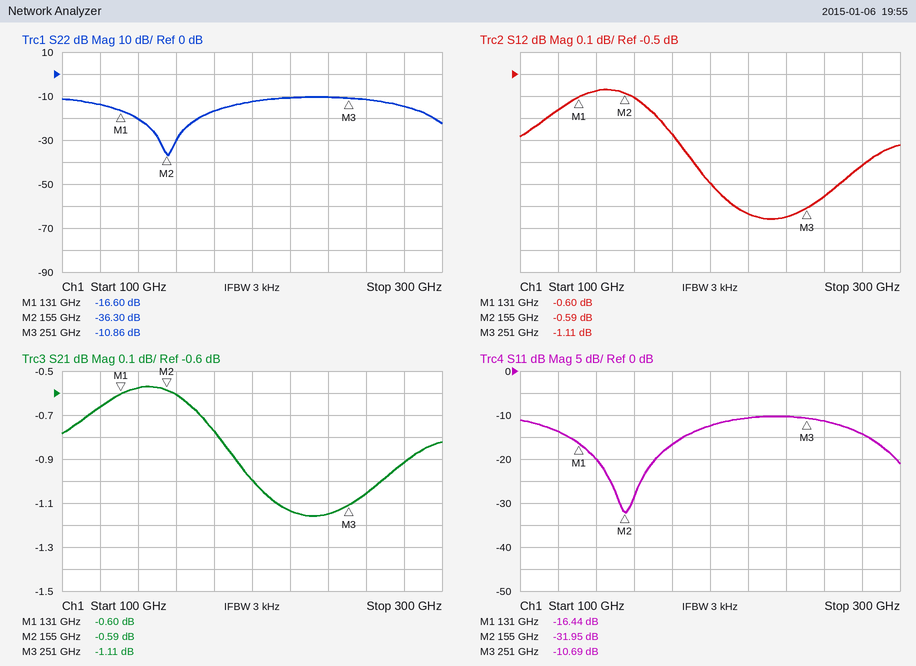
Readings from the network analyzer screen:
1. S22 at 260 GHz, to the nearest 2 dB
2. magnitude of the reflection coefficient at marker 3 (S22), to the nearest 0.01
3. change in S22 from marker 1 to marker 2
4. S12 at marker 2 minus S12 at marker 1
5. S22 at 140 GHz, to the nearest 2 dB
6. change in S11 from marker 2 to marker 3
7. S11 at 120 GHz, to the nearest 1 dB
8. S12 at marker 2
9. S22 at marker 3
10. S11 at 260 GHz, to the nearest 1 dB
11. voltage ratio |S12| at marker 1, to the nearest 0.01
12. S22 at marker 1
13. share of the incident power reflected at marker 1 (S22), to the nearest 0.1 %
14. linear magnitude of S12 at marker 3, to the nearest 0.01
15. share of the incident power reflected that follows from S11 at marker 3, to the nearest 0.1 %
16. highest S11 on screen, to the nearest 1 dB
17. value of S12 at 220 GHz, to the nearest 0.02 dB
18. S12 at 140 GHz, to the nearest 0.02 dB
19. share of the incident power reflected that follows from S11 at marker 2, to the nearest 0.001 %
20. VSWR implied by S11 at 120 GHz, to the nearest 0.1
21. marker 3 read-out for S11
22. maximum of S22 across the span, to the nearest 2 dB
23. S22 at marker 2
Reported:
-12 dB
0.29
-19.70 dB
0.01 dB
-20 dB
21.26 dB
-14 dB
-0.59 dB
-10.86 dB
-11 dB
0.93
-16.60 dB
2.2 %
0.88
8.5 %
-10 dB
-1.14 dB
-0.58 dB
0.064 %
1.5
-10.69 dB
-10 dB
-36.30 dB
